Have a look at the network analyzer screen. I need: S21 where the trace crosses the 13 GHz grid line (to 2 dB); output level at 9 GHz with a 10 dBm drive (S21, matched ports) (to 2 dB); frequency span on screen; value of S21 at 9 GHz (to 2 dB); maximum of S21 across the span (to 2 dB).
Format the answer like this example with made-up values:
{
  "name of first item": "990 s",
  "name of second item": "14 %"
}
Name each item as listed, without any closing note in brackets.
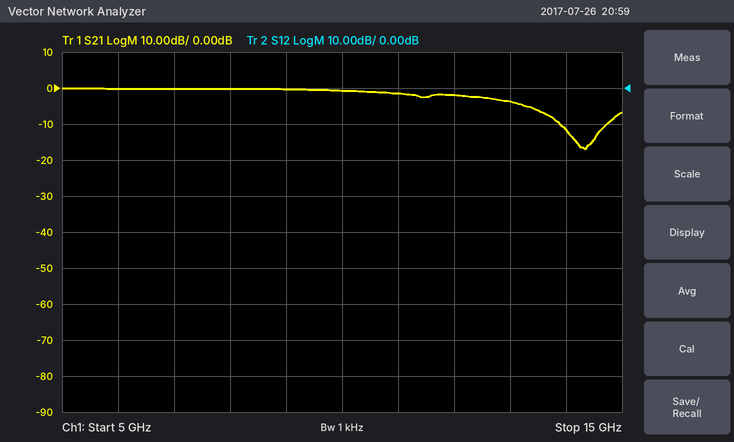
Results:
{
  "S21 where the trace crosses the 13 GHz grid line": "-4 dB",
  "output level at 9 GHz with a 10 dBm drive (S21, matched ports)": "10 dBm",
  "frequency span on screen": "10 GHz",
  "value of S21 at 9 GHz": "0 dB",
  "maximum of S21 across the span": "0 dB"
}
